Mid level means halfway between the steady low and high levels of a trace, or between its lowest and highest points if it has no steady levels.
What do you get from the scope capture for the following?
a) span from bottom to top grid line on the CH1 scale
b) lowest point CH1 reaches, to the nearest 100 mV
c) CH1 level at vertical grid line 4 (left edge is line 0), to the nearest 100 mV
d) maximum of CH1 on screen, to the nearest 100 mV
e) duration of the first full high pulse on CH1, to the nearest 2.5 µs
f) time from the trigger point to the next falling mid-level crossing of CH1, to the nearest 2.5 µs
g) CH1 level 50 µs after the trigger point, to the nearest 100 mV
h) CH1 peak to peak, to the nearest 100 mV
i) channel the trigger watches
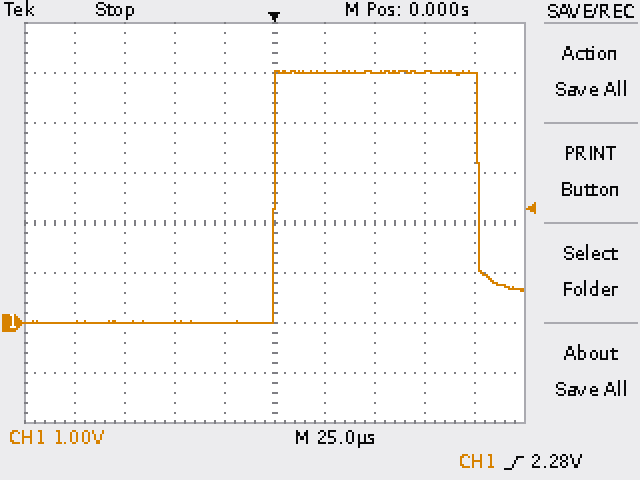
8 V
0.0 V
0.0 V
5.0 V
102.5 µs
102.5 µs
5.0 V
5.0 V
CH1
